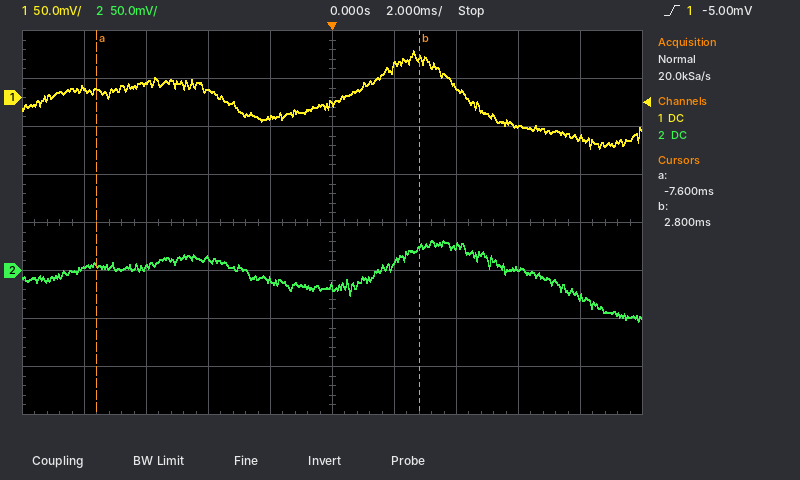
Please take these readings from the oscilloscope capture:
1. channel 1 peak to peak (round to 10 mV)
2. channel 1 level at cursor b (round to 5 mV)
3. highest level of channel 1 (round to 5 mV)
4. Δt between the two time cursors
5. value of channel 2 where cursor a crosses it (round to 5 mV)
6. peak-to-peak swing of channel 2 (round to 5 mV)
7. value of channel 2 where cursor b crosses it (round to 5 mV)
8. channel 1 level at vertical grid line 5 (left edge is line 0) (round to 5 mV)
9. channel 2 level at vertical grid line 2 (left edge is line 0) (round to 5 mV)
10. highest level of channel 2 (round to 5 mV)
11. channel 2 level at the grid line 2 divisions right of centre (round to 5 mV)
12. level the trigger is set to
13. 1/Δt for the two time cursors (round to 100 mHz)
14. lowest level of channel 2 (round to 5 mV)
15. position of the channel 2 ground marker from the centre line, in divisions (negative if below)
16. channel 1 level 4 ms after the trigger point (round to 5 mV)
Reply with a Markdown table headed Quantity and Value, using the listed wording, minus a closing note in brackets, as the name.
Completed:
| Quantity | Value |
|---|---|
| channel 1 peak to peak | 100 mV |
| channel 1 level at cursor b | 40 mV |
| highest level of channel 1 | 50 mV |
| Δt between the two time cursors | 10.4 ms |
| value of channel 2 where cursor a crosses it | 5 mV |
| peak-to-peak swing of channel 2 | 85 mV |
| value of channel 2 where cursor b crosses it | 25 mV |
| channel 1 level at vertical grid line 5 (left edge is line 0) | -5 mV |
| channel 2 level at vertical grid line 2 (left edge is line 0) | 5 mV |
| highest level of channel 2 | 30 mV |
| channel 2 level at the grid line 2 divisions right of centre | 25 mV |
| level the trigger is set to | -5.00 mV |
| 1/Δt for the two time cursors | 96.2 Hz |
| lowest level of channel 2 | -55 mV |
| position of the channel 2 ground marker from the centre line, in divisions | -1.0 div |
| channel 1 level 4 ms after the trigger point | 10 mV |
